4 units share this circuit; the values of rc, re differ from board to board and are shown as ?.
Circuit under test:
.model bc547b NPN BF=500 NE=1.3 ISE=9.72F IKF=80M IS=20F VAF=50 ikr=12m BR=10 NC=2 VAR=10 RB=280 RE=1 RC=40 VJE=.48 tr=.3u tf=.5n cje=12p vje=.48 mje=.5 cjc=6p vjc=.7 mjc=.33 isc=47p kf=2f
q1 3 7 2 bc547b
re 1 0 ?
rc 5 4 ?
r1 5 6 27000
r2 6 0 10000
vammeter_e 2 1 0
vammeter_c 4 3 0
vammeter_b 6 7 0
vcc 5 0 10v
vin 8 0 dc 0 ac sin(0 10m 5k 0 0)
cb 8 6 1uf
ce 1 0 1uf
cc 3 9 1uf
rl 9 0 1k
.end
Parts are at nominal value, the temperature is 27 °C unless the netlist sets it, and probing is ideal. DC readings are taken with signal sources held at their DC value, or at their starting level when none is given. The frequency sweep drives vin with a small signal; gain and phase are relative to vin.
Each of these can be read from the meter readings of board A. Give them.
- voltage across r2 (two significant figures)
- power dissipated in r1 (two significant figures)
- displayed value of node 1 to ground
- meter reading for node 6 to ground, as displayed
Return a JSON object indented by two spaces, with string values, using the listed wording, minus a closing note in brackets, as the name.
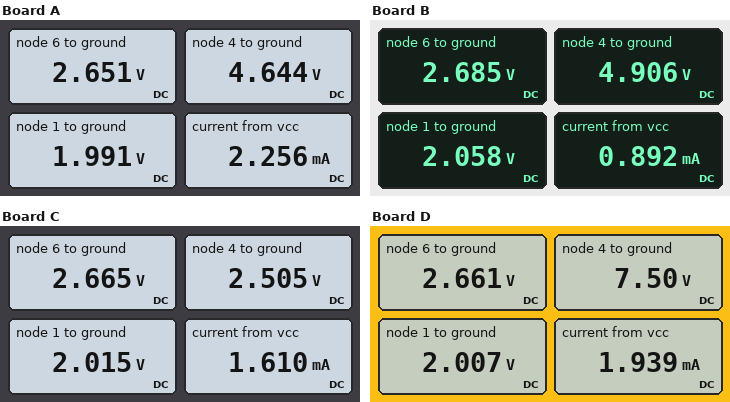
{
  "voltage across r2": "2.7 V",
  "power dissipated in r1": "2.0 mW",
  "displayed value of node 1 to ground": "1.991 V",
  "meter reading for node 6 to ground, as displayed": "2.651 V"
}
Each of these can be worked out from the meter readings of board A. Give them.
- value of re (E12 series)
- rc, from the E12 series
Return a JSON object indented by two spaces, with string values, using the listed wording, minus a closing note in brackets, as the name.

{
  "value of re": "1 kΩ",
  "rc, from the E12 series": "2.7 kΩ"
}
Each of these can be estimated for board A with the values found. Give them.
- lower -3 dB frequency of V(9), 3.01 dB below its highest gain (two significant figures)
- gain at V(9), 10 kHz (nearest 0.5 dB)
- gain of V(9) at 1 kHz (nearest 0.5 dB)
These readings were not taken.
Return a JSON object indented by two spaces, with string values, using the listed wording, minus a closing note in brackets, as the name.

{
  "lower -3 dB frequency of V(9), 3.01 dB below its highest gain": "10 kHz",
  "gain at V(9), 10 kHz": "30.0 dB",
  "gain of V(9) at 1 kHz": "13.0 dB"
}
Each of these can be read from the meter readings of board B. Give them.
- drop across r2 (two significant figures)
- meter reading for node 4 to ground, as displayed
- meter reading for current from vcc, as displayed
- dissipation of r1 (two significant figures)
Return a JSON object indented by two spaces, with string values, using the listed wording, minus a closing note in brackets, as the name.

{
  "drop across r2": "2.7 V",
  "meter reading for node 4 to ground, as displayed": "4.906 V",
  "meter reading for current from vcc, as displayed": "0.892 mA",
  "dissipation of r1": "2.0 mW"
}
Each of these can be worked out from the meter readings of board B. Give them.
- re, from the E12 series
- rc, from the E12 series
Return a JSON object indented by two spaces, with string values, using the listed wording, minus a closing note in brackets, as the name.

{
  "re, from the E12 series": "3.3 kΩ",
  "rc, from the E12 series": "8.2 kΩ"
}
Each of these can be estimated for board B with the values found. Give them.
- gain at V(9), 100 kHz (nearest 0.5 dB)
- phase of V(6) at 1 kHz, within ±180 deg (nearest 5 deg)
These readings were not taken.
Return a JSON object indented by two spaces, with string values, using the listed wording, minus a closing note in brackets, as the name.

{
  "gain at V(9), 100 kHz": "26.0 dB",
  "phase of V(6) at 1 kHz, within ±180 deg": "0 deg"
}
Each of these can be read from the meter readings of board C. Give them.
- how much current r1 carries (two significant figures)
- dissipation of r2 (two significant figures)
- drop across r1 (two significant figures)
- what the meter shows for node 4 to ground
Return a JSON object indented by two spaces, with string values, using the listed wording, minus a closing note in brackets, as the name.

{
  "how much current r1 carries": "270 µA",
  "dissipation of r2": "710 µW",
  "drop across r1": "7.3 V",
  "what the meter shows for node 4 to ground": "2.505 V"
}
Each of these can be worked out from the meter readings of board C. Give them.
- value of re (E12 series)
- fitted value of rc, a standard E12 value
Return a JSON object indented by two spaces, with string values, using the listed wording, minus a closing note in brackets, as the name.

{
  "value of re": "1.5 kΩ",
  "fitted value of rc, a standard E12 value": "5.6 kΩ"
}
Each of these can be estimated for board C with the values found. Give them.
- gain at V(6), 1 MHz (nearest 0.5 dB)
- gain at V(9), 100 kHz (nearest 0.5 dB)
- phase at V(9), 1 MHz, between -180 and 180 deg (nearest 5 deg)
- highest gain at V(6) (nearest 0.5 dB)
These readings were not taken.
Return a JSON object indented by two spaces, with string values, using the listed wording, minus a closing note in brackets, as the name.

{
  "gain at V(6), 1 MHz": "0 dB",
  "gain at V(9), 100 kHz": "31.5 dB",
  "phase at V(9), 1 MHz, between -180 and 180 deg": "150 deg",
  "highest gain at V(6)": "0 dB"
}
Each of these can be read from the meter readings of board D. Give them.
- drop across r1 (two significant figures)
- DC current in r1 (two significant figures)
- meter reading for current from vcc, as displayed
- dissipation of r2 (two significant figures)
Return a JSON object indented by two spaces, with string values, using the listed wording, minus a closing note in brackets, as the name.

{
  "drop across r1": "7.3 V",
  "DC current in r1": "270 µA",
  "meter reading for current from vcc, as displayed": "1.939 mA",
  "dissipation of r2": "710 µW"
}
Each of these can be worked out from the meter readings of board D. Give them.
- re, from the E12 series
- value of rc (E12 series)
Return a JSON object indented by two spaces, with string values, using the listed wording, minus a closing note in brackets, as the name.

{
  "re, from the E12 series": "1.2 kΩ",
  "value of rc": "1.5 kΩ"
}
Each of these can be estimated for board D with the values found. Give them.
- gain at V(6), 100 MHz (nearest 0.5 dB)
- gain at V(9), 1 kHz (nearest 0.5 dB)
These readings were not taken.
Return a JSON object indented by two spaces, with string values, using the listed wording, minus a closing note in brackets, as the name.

{
  "gain at V(6), 100 MHz": "0 dB",
  "gain at V(9), 1 kHz": "11.5 dB"
}
